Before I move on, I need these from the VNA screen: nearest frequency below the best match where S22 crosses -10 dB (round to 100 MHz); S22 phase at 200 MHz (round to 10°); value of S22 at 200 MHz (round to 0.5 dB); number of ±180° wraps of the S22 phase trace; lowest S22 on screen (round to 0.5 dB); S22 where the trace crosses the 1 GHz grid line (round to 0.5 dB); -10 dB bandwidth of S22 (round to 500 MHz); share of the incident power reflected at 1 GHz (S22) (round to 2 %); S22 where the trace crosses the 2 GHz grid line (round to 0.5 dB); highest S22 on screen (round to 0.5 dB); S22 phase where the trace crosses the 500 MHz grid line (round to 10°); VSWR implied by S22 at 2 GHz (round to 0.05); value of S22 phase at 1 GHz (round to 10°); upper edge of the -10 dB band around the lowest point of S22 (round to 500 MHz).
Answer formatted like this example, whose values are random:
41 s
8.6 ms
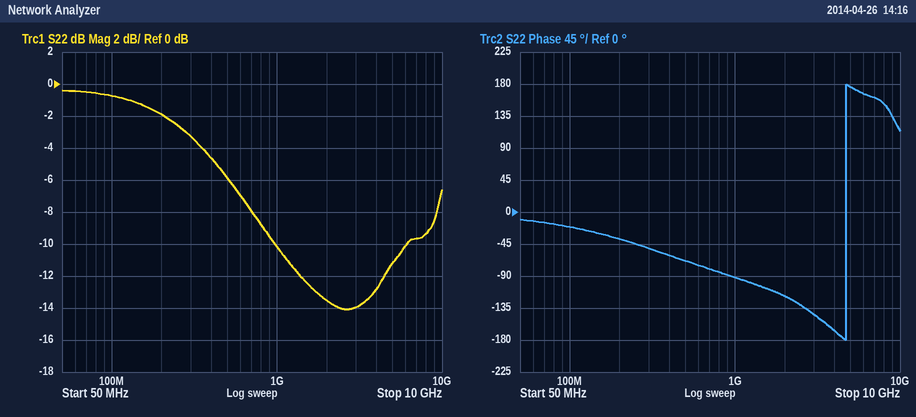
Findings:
1.0 GHz
-40°
-2.0 dB
1
-14.0 dB
-10.0 dB
5.0 GHz
10 %
-13.5 dB
-0.5 dB
-70°
1.55
-90°
6.0 GHz
